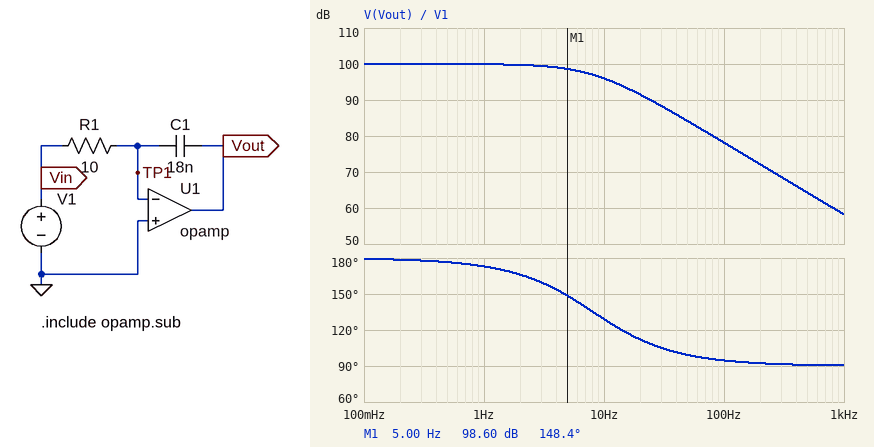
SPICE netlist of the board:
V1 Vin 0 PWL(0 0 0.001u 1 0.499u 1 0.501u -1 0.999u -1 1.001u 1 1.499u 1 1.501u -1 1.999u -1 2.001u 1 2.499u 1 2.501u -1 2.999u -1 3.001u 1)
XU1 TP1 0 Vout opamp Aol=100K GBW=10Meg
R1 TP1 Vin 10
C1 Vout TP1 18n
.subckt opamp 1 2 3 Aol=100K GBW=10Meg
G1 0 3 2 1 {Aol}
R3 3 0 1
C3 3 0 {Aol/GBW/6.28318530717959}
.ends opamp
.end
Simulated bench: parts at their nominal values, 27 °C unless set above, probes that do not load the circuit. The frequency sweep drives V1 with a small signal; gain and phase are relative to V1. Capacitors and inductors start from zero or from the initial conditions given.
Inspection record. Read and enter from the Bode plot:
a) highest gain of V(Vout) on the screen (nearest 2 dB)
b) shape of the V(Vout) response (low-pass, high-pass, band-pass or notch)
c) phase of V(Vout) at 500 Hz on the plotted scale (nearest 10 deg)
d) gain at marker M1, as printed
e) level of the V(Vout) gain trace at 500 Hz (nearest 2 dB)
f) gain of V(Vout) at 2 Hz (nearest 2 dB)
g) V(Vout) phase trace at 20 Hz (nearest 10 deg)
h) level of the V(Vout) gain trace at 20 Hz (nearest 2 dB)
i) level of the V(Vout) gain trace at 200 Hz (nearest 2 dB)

100 dB
low-pass
90 deg
98.60 dB
64 dB
100 dB
110 deg
92 dB
72 dB
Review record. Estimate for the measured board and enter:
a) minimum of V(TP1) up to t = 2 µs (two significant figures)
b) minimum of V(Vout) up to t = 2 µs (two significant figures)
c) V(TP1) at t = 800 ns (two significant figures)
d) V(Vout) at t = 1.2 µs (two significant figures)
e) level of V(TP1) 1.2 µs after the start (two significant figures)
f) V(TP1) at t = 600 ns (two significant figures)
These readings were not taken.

-81 mV
-2.5 V
-81 mV
-940 mV
81 mV
-81 mV
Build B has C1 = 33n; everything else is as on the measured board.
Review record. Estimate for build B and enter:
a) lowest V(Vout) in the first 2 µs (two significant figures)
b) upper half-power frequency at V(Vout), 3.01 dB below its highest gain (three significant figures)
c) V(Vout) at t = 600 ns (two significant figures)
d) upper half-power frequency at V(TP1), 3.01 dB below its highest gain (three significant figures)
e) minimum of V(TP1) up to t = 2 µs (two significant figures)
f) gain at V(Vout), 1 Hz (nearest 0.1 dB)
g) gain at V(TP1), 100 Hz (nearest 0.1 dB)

-1.4 V
4.60 Hz
-1.2 V
4.61 Hz
-46 mV
99.8 dB
-23.7 dB
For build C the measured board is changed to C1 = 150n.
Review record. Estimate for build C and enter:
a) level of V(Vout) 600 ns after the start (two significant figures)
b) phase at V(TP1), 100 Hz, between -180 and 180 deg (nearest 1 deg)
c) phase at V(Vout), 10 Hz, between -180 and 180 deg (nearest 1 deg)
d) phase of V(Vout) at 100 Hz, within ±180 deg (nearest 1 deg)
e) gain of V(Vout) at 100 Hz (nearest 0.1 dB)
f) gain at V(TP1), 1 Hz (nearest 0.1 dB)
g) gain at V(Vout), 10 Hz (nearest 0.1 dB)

-270 mV
-44 deg
96 deg
91 deg
60.4 dB
-2.8 dB
80.4 dB
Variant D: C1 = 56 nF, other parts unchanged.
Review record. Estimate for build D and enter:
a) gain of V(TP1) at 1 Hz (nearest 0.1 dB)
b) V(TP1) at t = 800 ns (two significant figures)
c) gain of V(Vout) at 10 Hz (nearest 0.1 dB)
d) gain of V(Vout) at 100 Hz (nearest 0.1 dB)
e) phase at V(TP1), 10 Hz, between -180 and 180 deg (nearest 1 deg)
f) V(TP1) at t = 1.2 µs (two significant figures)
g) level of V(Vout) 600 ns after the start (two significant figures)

-0.5 dB
-28 mV
88.5 dB
68.8 dB
-69 deg
28 mV
-720 mV
